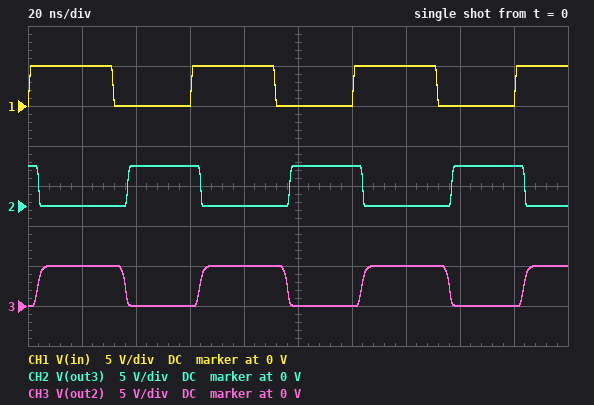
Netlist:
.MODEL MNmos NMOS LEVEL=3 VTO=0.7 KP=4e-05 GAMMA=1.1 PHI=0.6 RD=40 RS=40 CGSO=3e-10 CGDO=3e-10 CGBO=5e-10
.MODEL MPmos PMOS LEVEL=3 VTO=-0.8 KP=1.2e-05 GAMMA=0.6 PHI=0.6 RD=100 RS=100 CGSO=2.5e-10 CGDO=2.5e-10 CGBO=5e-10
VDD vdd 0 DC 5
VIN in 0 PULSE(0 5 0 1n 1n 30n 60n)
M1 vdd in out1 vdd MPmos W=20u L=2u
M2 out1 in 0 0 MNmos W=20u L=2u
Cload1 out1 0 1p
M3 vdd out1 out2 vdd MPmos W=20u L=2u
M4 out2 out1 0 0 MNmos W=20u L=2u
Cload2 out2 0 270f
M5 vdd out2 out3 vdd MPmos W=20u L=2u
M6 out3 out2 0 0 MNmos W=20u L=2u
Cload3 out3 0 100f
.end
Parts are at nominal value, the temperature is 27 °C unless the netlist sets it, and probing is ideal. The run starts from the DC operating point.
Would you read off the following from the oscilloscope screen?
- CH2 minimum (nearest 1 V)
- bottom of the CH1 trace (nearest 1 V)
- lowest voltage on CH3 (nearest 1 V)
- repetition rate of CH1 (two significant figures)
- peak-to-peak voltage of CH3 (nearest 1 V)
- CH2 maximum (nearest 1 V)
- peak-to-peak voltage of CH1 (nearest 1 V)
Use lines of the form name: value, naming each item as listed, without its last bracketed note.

CH2 minimum: 0 V
bottom of the CH1 trace: 0 V
lowest voltage on CH3: 0 V
repetition rate of CH1: 17 MHz
peak-to-peak voltage of CH3: 5 V
CH2 maximum: 5 V
peak-to-peak voltage of CH1: 5 V
